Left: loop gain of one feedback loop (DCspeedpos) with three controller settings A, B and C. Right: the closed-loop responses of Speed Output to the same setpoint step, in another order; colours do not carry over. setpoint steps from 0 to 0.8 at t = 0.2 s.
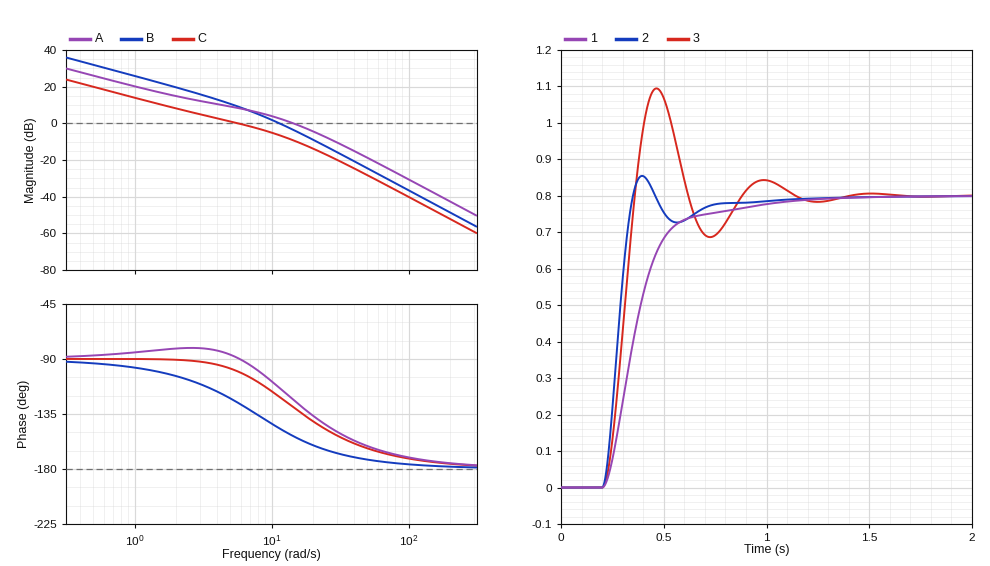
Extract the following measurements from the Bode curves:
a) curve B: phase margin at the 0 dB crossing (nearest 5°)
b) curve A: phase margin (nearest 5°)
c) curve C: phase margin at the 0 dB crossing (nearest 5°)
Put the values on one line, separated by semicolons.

35°; 55°; 80°
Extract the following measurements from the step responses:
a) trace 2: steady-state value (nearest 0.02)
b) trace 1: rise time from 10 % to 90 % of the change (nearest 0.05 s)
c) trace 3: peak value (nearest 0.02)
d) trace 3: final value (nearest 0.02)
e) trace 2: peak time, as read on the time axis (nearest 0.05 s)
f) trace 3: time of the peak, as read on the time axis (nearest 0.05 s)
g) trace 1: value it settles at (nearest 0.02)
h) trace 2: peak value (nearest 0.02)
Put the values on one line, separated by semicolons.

0.80; 0.30 s; 1.10; 0.80; 0.40 s; 0.45 s; 0.80; 0.86
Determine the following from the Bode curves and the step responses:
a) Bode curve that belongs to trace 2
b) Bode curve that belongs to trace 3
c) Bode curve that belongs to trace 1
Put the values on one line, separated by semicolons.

A; B; C
